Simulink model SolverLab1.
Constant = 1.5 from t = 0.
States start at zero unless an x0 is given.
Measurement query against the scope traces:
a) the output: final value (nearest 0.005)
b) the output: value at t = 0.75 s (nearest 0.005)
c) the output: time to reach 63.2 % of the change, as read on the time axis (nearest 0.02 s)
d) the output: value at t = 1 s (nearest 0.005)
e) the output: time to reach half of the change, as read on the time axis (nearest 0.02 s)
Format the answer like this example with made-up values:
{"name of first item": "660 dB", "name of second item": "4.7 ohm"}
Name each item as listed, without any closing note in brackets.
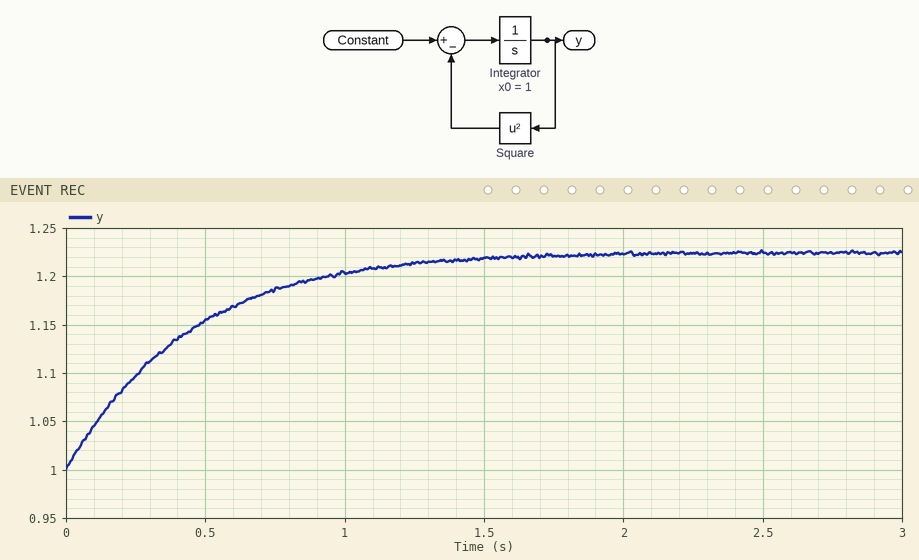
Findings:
{"the output: final value": "1.225", "the output: value at t = 0.75 s": "1.185", "the output: time to reach 63.2 % of the change, as read on the time axis": "0.44 s", "the output: value at t = 1 s": "1.205", "the output: time to reach half of the change, as read on the time axis": "0.30 s"}
